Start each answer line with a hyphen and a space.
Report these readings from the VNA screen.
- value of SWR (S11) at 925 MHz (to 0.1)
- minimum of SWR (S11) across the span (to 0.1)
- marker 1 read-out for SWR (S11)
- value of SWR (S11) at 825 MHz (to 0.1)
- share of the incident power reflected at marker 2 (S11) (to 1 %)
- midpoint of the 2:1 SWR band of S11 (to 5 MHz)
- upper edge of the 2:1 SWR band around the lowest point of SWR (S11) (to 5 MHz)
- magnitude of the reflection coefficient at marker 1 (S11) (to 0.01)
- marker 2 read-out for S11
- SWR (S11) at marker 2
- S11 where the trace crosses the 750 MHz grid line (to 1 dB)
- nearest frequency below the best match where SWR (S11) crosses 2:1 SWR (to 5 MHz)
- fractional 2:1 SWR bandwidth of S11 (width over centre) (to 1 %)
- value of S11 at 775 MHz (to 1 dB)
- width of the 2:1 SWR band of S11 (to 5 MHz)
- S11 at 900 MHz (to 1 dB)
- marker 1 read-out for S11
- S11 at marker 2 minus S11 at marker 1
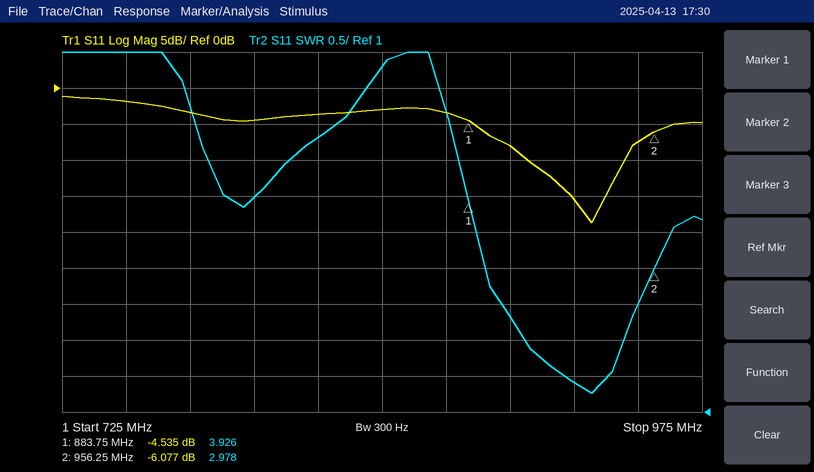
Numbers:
- 1.4
- 1.3
- 3.926
- 4.8
- 25 %
- 925 MHz
- 945 MHz
- 0.59
- -6.077 dB
- 2.978
- -2 dB
- 905 MHz
- 4 %
- -3 dB
- 40 MHz
- -8 dB
- -4.535 dB
- -1.542 dB
